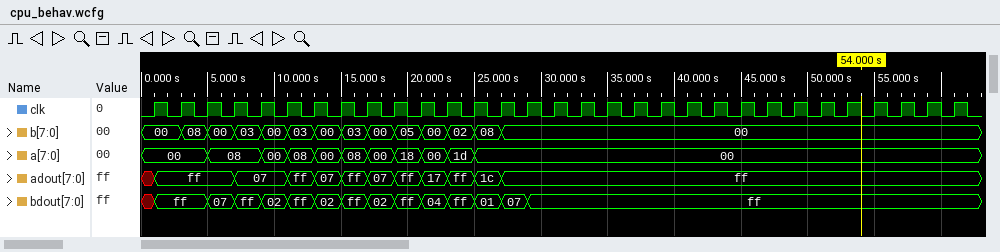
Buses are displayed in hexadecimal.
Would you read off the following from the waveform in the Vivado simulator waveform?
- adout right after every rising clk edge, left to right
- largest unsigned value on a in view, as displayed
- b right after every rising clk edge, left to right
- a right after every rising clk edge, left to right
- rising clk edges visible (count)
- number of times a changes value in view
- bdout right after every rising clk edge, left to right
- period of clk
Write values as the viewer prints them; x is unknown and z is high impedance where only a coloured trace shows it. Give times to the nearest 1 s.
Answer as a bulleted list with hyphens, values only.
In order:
- ff, ff, ff, 07, 07, ff, 07, ff, 07, ff, 17, ff, 1c, ff, ff, ff, ff, ff, ff, ff, ff, ff, ff, ff, ff, ff, ff, ff, ff, ff, ff
- 1d
- 00, 08, 00, 03, 00, 03, 00, 03, 00, 05, 00, 02, 08, 00, 00, 00, 00, 00, 00, 00, 00, 00, 00, 00, 00, 00, 00, 00, 00, 00, 00
- 00, 00, 08, 08, 00, 08, 00, 08, 00, 18, 00, 1d, 00, 00, 00, 00, 00, 00, 00, 00, 00, 00, 00, 00, 00, 00, 00, 00, 00, 00, 00
- 31
- 10
- ff, ff, 07, ff, 02, ff, 02, ff, 02, ff, 04, ff, 01, 07, ff, ff, ff, ff, ff, ff, ff, ff, ff, ff, ff, ff, ff, ff, ff, ff, ff
- 2 s
